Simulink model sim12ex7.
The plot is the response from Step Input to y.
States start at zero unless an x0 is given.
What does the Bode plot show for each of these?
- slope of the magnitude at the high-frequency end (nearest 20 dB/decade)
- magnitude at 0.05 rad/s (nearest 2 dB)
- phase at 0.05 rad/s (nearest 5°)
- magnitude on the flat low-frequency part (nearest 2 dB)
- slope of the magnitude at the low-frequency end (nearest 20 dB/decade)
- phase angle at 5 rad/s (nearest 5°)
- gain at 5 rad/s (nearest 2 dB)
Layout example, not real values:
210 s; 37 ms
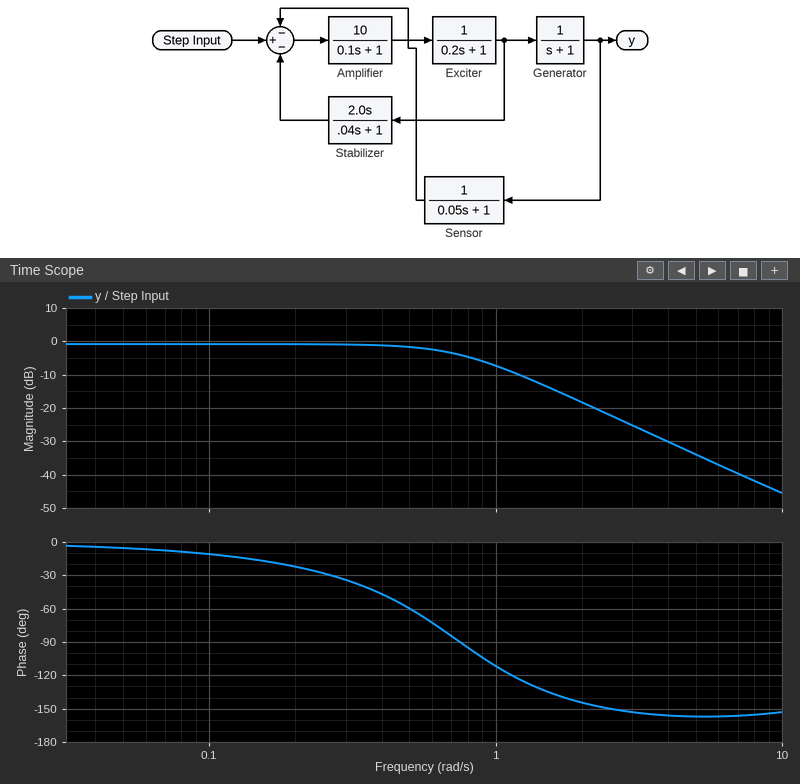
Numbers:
-40 dB/decade; 0 dB; -5°; 0 dB; 0 dB/decade; -155°; -34 dB
